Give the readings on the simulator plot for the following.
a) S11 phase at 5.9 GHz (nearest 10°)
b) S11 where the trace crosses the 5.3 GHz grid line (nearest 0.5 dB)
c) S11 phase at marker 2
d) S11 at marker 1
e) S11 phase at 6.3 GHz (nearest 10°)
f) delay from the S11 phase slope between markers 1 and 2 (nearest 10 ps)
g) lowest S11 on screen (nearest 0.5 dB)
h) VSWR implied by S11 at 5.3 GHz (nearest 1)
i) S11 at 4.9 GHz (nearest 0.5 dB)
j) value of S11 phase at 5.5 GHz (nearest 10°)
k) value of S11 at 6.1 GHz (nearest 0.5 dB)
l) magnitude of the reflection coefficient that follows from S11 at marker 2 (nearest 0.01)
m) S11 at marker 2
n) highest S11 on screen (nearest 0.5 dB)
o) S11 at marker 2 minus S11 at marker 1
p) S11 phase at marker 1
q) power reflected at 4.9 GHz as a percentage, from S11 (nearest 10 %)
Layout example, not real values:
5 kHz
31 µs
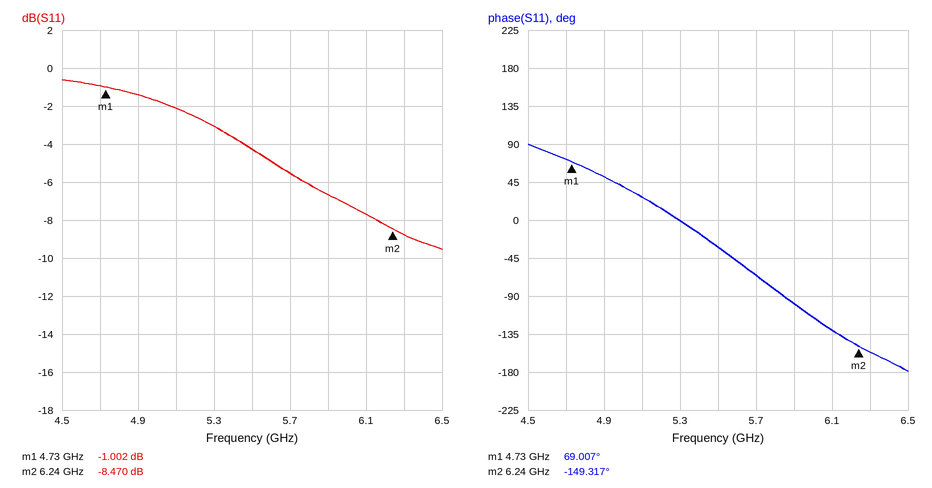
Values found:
-100°
-3.0 dB
-149.317°
-1.002 dB
-160°
400 ps
-9.5 dB
6
-1.5 dB
-30°
-7.5 dB
0.38
-8.470 dB
-0.5 dB
-7.468 dB
69.007°
70 %
